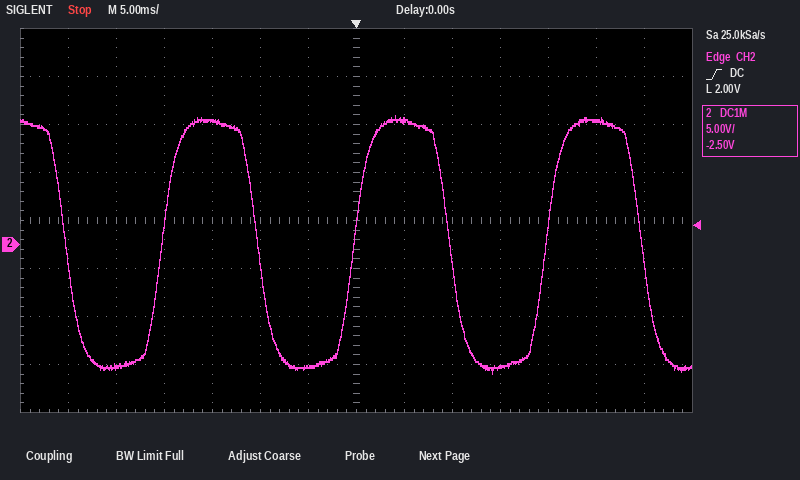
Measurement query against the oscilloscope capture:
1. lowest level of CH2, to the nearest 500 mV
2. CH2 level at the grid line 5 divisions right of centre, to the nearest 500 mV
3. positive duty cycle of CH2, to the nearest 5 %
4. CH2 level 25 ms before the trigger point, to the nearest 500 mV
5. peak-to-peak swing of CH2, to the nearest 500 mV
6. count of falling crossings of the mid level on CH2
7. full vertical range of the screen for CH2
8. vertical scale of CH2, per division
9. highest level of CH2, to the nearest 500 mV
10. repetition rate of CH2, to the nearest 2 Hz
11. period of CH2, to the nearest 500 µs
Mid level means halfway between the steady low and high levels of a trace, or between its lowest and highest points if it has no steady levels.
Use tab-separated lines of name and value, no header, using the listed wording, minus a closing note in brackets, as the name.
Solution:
lowest level of CH2, to the nearest 500 mV	-13.5 V
CH2 level at the grid line 5 divisions right of centre, to the nearest 500 mV	13.0 V
positive duty cycle of CH2, to the nearest 5 %	50 %
CH2 level 25 ms before the trigger point, to the nearest 500 mV	-12.5 V
peak-to-peak swing of CH2, to the nearest 500 mV	27.0 V
count of falling crossings of the mid level on CH2	4
full vertical range of the screen for CH2	40 V
vertical scale of CH2, per division	5 V
highest level of CH2, to the nearest 500 mV	13.5 V
repetition rate of CH2, to the nearest 2 Hz	50 Hz
period of CH2, to the nearest 500 µs	20.0 ms
